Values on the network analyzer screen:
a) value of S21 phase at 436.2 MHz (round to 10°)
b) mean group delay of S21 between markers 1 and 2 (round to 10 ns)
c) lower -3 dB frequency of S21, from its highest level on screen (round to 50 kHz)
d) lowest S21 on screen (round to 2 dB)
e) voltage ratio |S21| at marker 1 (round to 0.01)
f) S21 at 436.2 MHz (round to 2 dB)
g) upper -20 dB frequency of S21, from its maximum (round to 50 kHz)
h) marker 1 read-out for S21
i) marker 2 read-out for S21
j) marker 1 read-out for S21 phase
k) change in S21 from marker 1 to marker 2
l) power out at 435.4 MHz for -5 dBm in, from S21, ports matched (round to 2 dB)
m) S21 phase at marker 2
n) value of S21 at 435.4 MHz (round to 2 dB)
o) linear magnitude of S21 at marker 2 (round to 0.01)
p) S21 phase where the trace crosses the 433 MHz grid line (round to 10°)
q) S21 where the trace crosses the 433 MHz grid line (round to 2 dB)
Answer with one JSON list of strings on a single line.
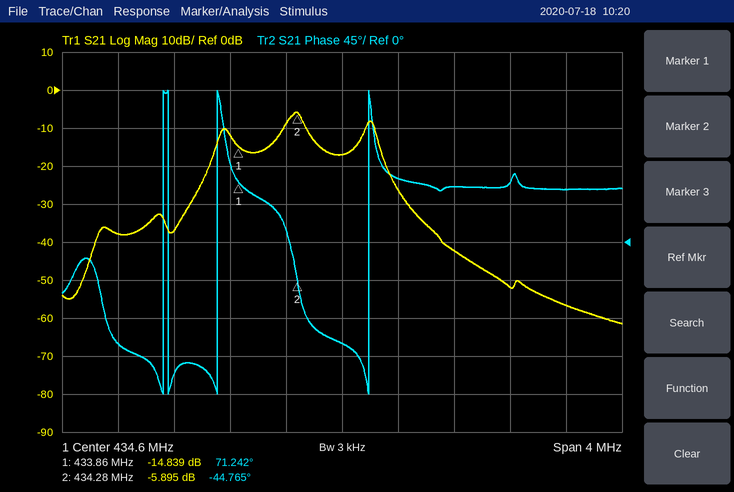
["60°", "770 ns", "434.20 MHz", "-62 dB", "0.18", "-56 dB", "435.00 MHz", "-14.839 dB", "-5.895 dB", "71.242°", "8.944 dB", "-48 dBm", "-44.765°", "-42 dB", "0.51", "-120°", "-38 dB"]
